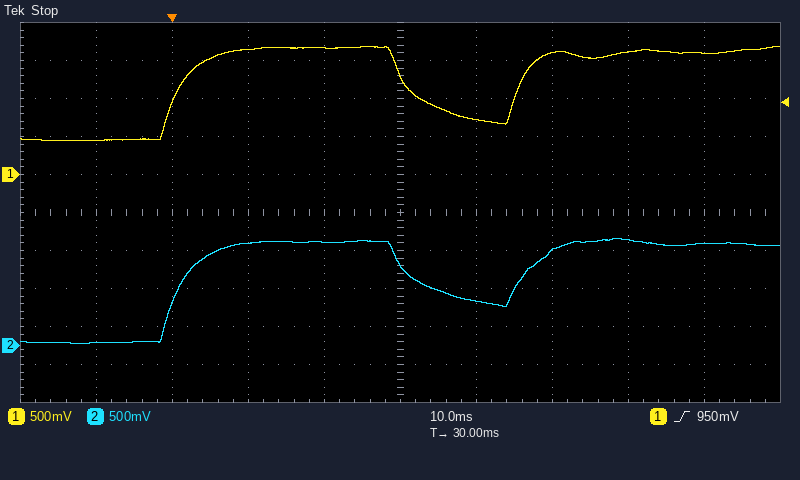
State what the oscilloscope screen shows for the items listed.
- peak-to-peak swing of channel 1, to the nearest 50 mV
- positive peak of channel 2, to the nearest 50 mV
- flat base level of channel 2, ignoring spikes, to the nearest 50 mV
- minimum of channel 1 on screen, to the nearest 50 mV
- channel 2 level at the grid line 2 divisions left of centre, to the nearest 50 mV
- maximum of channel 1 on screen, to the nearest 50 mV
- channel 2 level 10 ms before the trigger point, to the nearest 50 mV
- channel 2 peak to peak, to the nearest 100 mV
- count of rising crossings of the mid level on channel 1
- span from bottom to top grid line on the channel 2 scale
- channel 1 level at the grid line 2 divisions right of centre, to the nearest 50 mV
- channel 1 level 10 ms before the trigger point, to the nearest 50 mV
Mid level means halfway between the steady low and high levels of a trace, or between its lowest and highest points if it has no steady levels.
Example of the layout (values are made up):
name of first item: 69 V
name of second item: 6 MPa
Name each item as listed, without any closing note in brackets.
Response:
peak-to-peak swing of channel 1, to the nearest 50 mV: 1.25 V
positive peak of channel 2, to the nearest 50 mV: 1.40 V
flat base level of channel 2, ignoring spikes, to the nearest 50 mV: 50 mV
minimum of channel 1 on screen, to the nearest 50 mV: 450 mV
channel 2 level at the grid line 2 divisions left of centre, to the nearest 50 mV: 1.35 V
maximum of channel 1 on screen, to the nearest 50 mV: 1.70 V
channel 2 level 10 ms before the trigger point, to the nearest 50 mV: 50 mV
channel 2 peak to peak, to the nearest 100 mV: 1.40 V
count of rising crossings of the mid level on channel 1: 2
span from bottom to top grid line on the channel 2 scale: 5 V
channel 1 level at the grid line 2 divisions right of centre, to the nearest 50 mV: 1.60 V
channel 1 level 10 ms before the trigger point, to the nearest 50 mV: 450 mV
